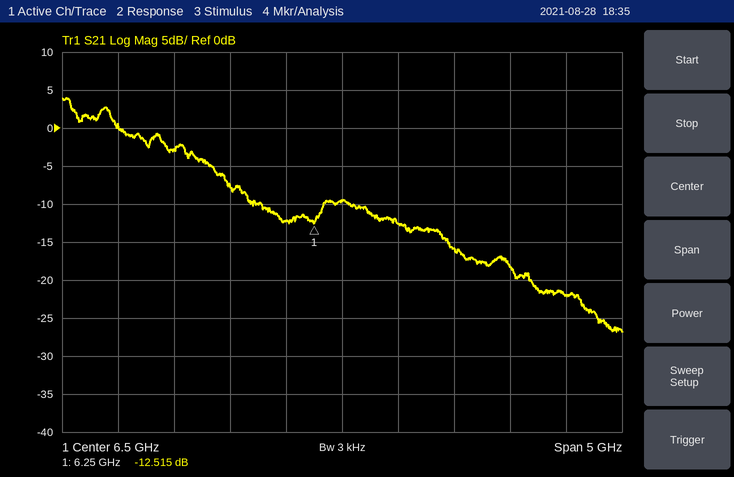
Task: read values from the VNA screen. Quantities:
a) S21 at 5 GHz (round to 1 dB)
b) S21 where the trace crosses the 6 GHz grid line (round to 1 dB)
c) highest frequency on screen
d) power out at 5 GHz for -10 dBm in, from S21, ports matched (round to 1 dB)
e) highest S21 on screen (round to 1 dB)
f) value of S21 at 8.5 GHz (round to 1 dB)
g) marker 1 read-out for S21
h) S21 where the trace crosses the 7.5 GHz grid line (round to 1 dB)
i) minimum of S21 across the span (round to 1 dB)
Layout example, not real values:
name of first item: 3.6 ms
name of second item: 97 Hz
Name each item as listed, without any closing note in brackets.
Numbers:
S21 at 5 GHz: -3 dB
S21 where the trace crosses the 6 GHz grid line: -12 dB
highest frequency on screen: 9 GHz
power out at 5 GHz for -10 dBm in, from S21, ports matched: -13 dBm
highest S21 on screen: 4 dB
value of S21 at 8.5 GHz: -22 dB
marker 1 read-out for S21: -12.515 dB
S21 where the trace crosses the 7.5 GHz grid line: -16 dB
minimum of S21 across the span: -27 dB
